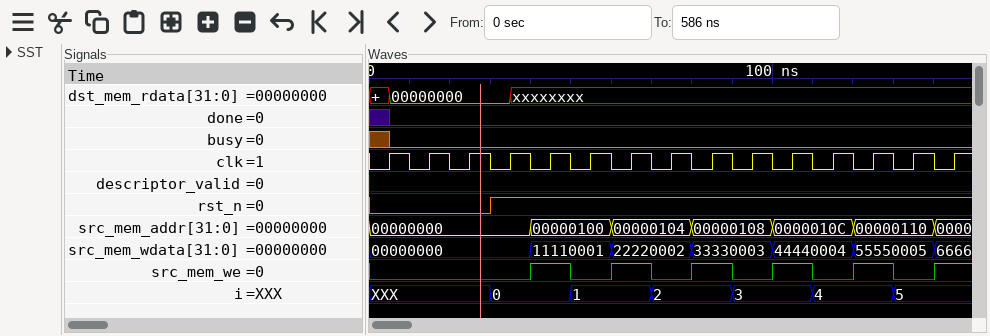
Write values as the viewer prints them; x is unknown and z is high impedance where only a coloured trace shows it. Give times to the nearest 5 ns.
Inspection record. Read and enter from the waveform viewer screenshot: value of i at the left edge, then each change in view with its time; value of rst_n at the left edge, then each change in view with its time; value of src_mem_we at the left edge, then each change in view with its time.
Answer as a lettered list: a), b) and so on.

a) XXX, 0 at 30 ns, 1 at 50 ns, 2 at 70 ns, 3 at 90 ns, 4 at 110 ns, 5 at 130 ns
b) 0, 1 at 30 ns
c) 0, 1 at 40 ns, 0 at 50 ns, 1 at 60 ns, 0 at 70 ns, 1 at 80 ns, 0 at 90 ns, 1 at 100 ns, 0 at 110 ns, 1 at 120 ns, 0 at 130 ns, 1 at 140 ns
